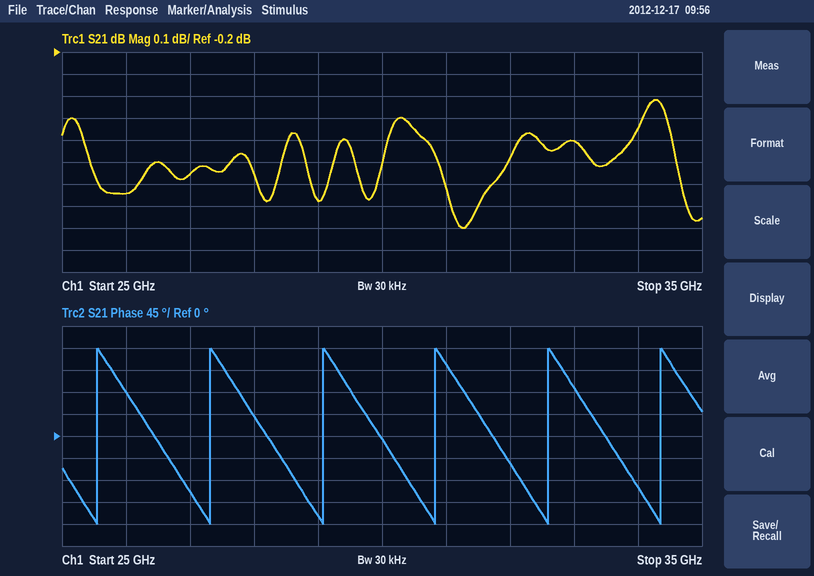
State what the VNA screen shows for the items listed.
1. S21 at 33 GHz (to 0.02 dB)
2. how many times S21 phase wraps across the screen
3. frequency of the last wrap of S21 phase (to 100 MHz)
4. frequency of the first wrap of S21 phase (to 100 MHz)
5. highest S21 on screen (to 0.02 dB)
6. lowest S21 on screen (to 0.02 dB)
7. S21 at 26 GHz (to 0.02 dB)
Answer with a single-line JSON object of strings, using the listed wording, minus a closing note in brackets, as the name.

{"S21 at 33 GHz": "-0.60 dB", "how many times S21 phase wraps across the screen": "6", "frequency of the last wrap of S21 phase": "34.4 GHz", "frequency of the first wrap of S21 phase": "25.5 GHz", "highest S21 on screen": "-0.42 dB", "lowest S21 on screen": "-1.00 dB", "S21 at 26 GHz": "-0.84 dB"}
